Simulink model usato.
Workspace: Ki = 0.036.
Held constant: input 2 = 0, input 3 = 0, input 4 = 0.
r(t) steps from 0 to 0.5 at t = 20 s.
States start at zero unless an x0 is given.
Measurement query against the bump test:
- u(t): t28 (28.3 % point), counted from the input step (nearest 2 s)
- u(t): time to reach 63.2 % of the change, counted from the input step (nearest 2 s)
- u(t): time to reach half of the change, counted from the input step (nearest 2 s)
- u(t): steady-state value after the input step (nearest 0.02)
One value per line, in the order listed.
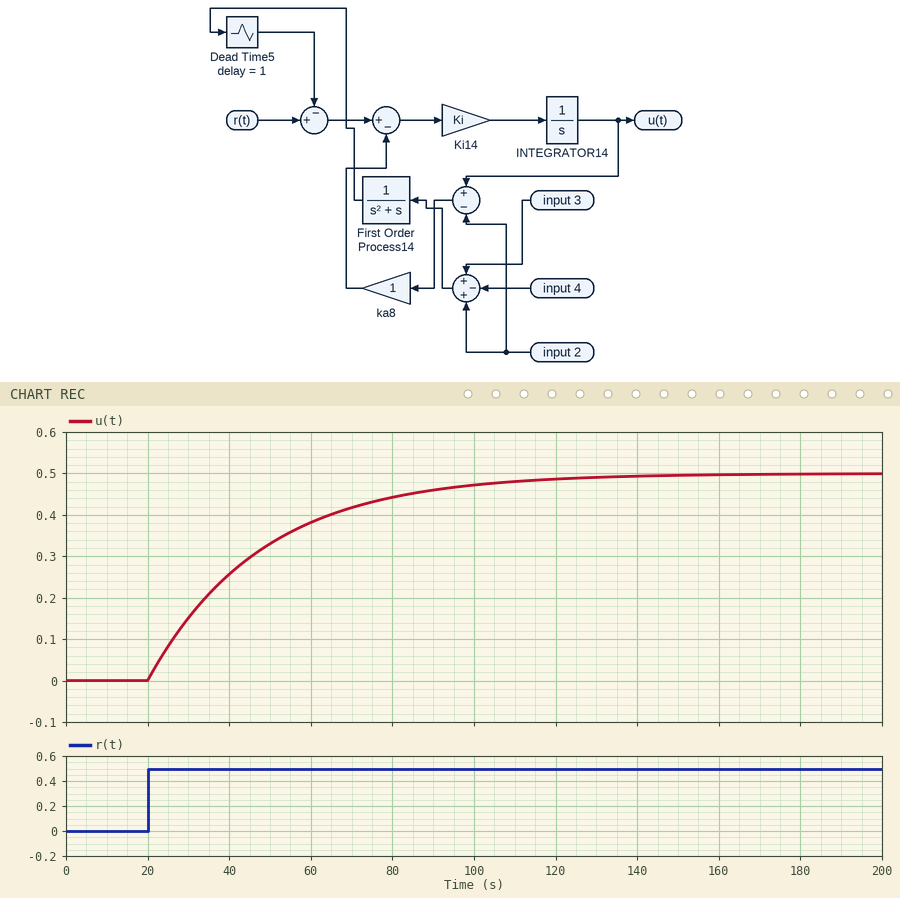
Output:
10 s
28 s
20 s
0.50
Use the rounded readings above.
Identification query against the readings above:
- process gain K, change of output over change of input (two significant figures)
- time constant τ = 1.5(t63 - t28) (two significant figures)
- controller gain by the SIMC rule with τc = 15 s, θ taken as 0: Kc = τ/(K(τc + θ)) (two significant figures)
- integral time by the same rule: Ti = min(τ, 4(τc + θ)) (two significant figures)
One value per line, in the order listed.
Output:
1.0
27 s
1.8
27 s
